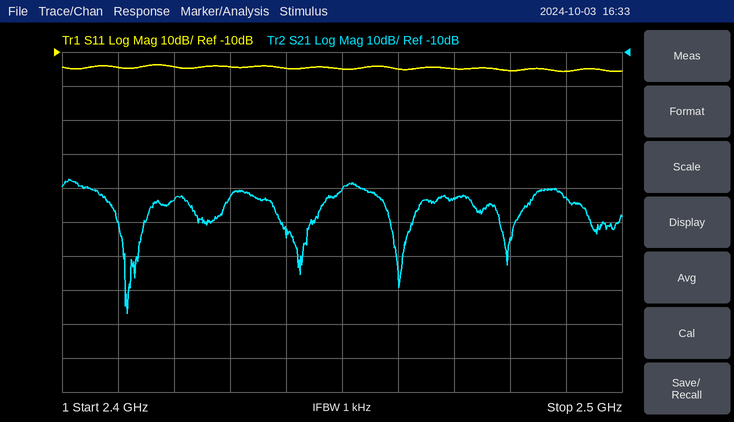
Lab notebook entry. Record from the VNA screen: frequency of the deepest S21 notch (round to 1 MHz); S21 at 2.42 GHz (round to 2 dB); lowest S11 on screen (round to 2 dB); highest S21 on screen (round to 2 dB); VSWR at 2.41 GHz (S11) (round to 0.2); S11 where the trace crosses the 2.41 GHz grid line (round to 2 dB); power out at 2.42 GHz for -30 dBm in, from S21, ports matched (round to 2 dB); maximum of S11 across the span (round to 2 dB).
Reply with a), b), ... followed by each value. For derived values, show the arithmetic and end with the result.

a) 2.412 GHz
b) -54 dB
c) -16 dB
d) -48 dB
e) |Γ| = 10^(-14/20) = 0.1995; VSWR = (1 + 0.1995)/(1 − 0.1995) ≈ 1.50, so 1.4 to the nearest 0.2
f) -14 dB
g) -30 dBm + (-54 dB) = -84 dBm
h) -14 dB
